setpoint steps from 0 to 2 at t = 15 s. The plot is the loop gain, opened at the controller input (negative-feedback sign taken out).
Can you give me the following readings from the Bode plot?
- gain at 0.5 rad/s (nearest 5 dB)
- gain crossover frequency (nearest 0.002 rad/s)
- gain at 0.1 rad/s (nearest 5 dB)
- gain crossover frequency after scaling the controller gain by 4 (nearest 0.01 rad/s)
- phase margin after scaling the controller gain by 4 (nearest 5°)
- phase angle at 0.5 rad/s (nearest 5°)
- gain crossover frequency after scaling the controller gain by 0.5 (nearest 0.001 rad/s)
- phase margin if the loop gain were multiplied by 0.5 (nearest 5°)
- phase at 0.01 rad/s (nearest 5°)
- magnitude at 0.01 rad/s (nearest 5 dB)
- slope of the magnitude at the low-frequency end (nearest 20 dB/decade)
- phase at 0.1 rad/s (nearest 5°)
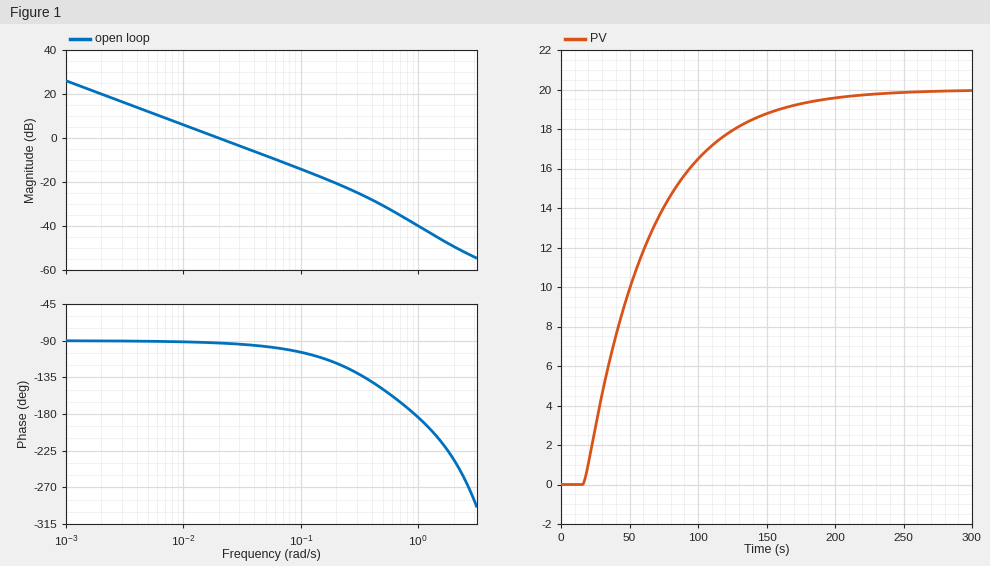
-30 dB
0.020 rad/s
-15 dB
0.08 rad/s
80°
-150°
0.010 rad/s
90°
-90°
5 dB
-20 dB/decade
-105°
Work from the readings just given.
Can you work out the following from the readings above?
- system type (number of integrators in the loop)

1
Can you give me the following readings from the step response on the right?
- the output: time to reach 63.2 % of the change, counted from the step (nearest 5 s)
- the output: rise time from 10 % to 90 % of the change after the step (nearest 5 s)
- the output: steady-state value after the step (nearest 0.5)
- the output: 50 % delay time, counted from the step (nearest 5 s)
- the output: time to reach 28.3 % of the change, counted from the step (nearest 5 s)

50 s
105 s
20.0
35 s
20 s
